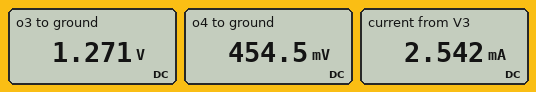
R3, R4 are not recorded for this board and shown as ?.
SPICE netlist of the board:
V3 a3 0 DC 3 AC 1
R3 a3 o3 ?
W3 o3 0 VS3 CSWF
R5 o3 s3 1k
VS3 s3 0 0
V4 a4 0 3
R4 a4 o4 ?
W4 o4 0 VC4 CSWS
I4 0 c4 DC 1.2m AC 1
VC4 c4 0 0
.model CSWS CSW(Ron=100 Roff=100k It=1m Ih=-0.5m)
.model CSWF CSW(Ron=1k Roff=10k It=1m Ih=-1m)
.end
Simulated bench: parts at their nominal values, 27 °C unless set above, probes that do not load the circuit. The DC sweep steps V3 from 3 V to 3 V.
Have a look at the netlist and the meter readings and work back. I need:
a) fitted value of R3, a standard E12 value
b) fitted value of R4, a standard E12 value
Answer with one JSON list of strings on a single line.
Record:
["680 Ω", "560 Ω"]
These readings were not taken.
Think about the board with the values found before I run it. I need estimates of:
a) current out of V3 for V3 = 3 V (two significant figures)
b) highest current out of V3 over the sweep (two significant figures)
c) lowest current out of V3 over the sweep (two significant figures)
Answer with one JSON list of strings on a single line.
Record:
["2.5 mA", "2.5 mA", "2.5 mA"]
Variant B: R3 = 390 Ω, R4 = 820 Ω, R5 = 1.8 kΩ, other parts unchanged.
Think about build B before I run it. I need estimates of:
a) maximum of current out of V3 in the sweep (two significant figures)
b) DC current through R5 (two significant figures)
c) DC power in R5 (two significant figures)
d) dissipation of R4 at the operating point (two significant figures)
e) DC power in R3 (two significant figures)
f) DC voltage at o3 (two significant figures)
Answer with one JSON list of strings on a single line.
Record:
["2.9 mA", "1.0 mA", "1.9 mW", "8.7 mW", "3.3 mW", "1.9 V"]
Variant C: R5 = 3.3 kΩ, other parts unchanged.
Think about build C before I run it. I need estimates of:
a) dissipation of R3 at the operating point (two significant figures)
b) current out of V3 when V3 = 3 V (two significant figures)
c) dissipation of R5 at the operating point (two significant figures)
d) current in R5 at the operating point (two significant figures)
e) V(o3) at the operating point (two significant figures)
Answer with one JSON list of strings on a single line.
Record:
["2.9 mW", "2.1 mA", "770 µW", "480 µA", "1.6 V"]
